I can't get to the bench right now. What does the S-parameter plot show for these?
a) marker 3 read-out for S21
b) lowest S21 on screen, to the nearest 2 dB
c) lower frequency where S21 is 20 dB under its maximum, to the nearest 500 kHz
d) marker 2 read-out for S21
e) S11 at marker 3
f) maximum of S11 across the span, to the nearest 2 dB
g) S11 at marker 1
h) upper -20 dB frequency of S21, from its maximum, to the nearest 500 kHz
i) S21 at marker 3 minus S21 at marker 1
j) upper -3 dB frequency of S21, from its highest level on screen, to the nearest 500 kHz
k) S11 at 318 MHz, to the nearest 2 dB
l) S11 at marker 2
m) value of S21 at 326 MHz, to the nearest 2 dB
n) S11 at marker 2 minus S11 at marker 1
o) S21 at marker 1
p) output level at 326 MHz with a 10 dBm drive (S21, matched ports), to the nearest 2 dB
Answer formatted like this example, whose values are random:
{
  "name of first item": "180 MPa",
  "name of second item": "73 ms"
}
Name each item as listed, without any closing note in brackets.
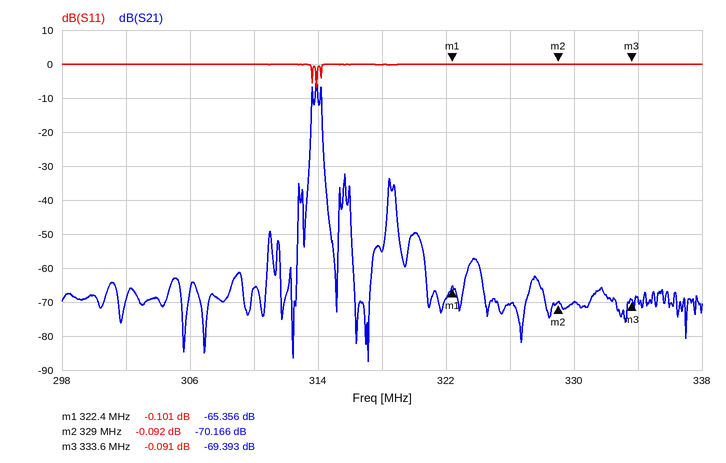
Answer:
{
  "marker 3 read-out for S21": "-69.393 dB",
  "lowest S21 on screen, to the nearest 2 dB": "-88 dB",
  "lower frequency where S21 is 20 dB under its maximum, to the nearest 500 kHz": "313.5 MHz",
  "marker 2 read-out for S21": "-70.166 dB",
  "S11 at marker 3": "-0.091 dB",
  "maximum of S11 across the span, to the nearest 2 dB": "0 dB",
  "S11 at marker 1": "-0.101 dB",
  "upper -20 dB frequency of S21, from its maximum, to the nearest 500 kHz": "314.5 MHz",
  "S21 at marker 3 minus S21 at marker 1": "-4.037 dB",
  "upper -3 dB frequency of S21, from its highest level on screen, to the nearest 500 kHz": "314.0 MHz",
  "S11 at 318 MHz, to the nearest 2 dB": "0 dB",
  "S11 at marker 2": "-0.092 dB",
  "value of S21 at 326 MHz, to the nearest 2 dB": "-70 dB",
  "S11 at marker 2 minus S11 at marker 1": "0.009 dB",
  "S21 at marker 1": "-65.356 dB",
  "output level at 326 MHz with a 10 dBm drive (S21, matched ports), to the nearest 2 dB": "-60 dBm"
}
